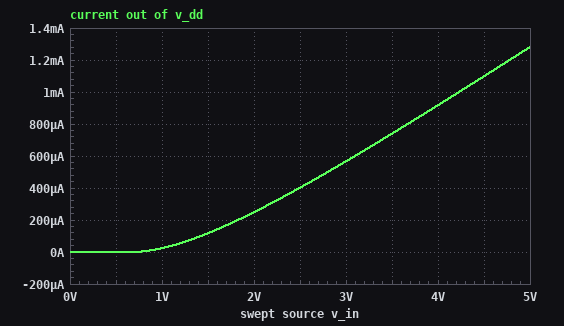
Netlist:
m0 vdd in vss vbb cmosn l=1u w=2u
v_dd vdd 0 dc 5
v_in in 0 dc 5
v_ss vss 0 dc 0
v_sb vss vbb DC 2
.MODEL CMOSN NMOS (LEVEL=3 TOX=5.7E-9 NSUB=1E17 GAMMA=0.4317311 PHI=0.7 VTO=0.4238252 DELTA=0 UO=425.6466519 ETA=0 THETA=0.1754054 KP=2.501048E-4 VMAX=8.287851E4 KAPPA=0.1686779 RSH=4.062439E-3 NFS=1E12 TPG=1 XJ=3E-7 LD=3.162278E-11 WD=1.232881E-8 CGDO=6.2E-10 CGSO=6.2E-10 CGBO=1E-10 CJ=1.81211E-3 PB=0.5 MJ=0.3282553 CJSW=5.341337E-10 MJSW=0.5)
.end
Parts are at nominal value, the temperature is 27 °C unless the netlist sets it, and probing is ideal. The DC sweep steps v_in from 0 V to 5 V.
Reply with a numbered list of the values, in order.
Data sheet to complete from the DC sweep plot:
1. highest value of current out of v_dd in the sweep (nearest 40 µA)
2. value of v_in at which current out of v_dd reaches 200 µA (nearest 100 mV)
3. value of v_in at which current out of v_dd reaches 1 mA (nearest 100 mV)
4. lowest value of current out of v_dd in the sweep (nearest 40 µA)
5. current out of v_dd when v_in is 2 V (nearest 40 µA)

1. 1.28 mA
2. 1.8 V
3. 4.2 V
4. 0 A
5. 240 µA
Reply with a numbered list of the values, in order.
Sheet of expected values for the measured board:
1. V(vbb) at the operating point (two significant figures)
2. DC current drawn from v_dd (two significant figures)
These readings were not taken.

1. -2.0 V
2. 1.3 mA
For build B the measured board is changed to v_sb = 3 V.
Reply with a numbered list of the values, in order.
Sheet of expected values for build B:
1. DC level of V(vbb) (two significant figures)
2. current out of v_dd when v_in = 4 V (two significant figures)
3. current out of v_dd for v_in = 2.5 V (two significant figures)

1. -3.0 V
2. 890 µA
3. 380 µA
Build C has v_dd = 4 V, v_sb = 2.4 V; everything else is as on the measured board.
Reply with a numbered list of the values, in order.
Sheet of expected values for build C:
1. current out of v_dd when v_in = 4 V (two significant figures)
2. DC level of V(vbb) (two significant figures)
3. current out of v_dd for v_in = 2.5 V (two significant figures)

1. 890 µA
2. -2.4 V
3. 390 µA
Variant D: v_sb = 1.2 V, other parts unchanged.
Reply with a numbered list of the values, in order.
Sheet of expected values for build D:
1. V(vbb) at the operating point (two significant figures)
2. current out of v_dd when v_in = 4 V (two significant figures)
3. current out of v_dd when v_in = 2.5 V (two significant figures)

1. -1.2 V
2. 940 µA
3. 430 µA
